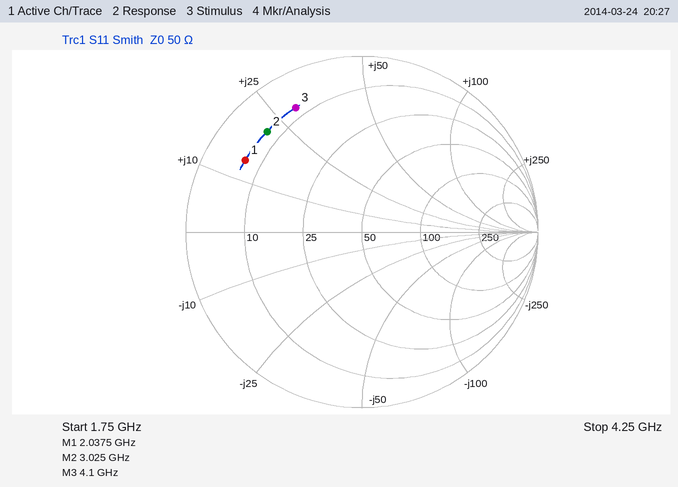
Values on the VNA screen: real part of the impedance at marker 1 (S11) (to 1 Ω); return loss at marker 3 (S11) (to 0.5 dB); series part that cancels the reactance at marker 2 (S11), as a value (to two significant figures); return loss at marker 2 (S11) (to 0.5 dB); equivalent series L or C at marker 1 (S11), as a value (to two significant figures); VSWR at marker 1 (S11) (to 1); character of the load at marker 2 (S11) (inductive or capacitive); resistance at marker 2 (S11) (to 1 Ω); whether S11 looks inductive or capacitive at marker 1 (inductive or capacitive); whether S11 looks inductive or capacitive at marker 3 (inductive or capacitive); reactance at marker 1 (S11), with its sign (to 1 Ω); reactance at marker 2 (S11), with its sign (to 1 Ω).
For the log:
7 Ω
2.0 dB
2.5 pF
2.0 dB
1.1 nH
8
inductive
7 Ω
inductive
inductive
+14 Ω
+21 Ω
